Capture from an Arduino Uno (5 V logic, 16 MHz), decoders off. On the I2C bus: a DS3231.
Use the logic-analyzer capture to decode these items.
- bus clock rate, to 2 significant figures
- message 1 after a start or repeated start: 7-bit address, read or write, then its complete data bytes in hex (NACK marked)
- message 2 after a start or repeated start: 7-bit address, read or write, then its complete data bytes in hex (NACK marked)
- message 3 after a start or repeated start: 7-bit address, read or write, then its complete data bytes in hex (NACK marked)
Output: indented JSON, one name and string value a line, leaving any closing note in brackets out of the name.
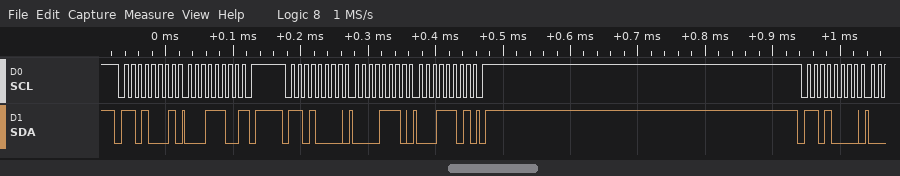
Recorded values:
{
  "bus clock rate, to 2 significant figures": "100 kHz",
  "message 1 after a start or repeated start: 7-bit address, read or write, then its complete data bytes in hex": "0x68 read: 1C NACK",
  "message 2 after a start or repeated start: 7-bit address, read or write, then its complete data bytes in hex": "0x68 write: 0E 1D",
  "message 3 after a start or repeated start: 7-bit address, read or write, then its complete data bytes in hex": "0x68 write"
}
